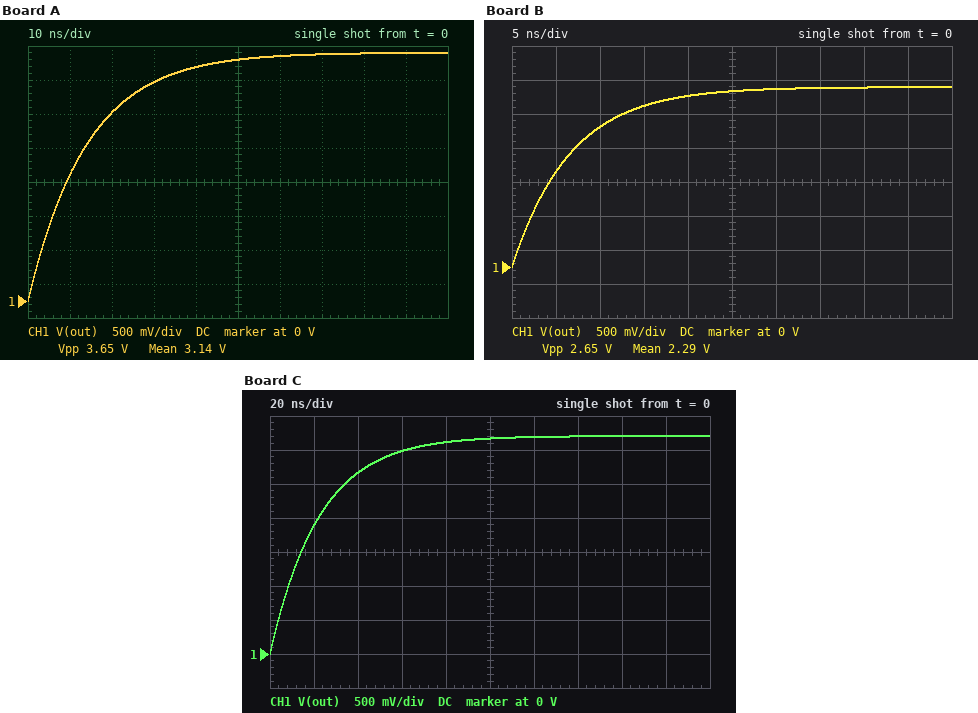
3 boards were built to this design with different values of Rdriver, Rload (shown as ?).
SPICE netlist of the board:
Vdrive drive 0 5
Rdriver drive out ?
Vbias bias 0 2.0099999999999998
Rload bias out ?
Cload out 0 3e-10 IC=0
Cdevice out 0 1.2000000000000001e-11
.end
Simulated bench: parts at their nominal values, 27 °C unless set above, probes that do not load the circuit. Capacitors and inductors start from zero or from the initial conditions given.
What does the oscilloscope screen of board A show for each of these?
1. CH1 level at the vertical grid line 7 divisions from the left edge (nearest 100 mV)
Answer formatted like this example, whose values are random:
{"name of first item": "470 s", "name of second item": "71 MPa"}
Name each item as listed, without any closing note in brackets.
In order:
{"CH1 level at the vertical grid line 7 divisions from the left edge": "3.6 V"}
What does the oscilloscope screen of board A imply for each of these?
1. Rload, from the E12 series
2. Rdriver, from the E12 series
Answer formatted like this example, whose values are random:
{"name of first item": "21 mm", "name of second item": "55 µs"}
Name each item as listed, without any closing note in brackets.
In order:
{"Rload, from the E12 series": "100 Ω", "Rdriver, from the E12 series": "82 Ω"}
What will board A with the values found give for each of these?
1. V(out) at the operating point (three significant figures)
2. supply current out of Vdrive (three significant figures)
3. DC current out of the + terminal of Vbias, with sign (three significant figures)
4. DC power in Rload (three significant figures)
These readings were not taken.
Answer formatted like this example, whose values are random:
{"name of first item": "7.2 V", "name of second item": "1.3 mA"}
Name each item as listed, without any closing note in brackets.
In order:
{"V(out) at the operating point": "3.65 V", "supply current out of Vdrive": "16.4 mA", "DC current out of the + terminal of Vbias, with sign": "-16.4 mA", "DC power in Rload": "27.0 mW"}
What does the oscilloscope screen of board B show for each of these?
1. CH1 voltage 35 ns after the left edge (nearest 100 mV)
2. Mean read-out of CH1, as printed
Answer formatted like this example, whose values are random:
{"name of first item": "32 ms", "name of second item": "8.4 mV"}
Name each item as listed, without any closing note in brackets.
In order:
{"CH1 voltage 35 ns after the left edge": "2.6 V", "Mean read-out of CH1, as printed": "2.29 V"}
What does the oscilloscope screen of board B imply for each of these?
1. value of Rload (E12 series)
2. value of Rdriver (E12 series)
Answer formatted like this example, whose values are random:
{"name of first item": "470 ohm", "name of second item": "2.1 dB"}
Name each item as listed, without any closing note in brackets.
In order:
{"value of Rload": "27 Ω", "value of Rdriver": "100 Ω"}
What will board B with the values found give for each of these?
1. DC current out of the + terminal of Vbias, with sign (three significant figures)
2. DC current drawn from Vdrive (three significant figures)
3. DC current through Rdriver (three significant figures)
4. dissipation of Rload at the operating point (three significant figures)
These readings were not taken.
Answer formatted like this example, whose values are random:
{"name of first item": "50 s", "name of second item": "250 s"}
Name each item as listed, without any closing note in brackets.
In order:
{"DC current out of the + terminal of Vbias, with sign": "-23.5 mA", "DC current drawn from Vdrive": "23.5 mA", "DC current through Rdriver": "23.5 mA", "dissipation of Rload at the operating point": "15.0 mW"}
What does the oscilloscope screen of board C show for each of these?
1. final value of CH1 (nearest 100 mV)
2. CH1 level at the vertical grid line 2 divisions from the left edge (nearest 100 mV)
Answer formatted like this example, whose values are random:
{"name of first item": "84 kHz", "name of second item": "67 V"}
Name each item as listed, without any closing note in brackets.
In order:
{"final value of CH1": "3.2 V", "CH1 level at the vertical grid line 2 divisions from the left edge": "2.7 V"}
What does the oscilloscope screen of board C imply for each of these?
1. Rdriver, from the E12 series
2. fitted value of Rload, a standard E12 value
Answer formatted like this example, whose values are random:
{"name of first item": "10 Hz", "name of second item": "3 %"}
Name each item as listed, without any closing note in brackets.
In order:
{"Rdriver, from the E12 series": "180 Ω", "fitted value of Rload, a standard E12 value": "120 Ω"}
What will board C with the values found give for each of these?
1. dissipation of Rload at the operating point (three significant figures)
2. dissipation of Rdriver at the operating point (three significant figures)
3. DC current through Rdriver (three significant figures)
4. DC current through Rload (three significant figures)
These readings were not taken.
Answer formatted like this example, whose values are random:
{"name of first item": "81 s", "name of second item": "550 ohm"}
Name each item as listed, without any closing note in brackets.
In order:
{"dissipation of Rload at the operating point": "11.9 mW", "dissipation of Rdriver at the operating point": "17.9 mW", "DC current through Rdriver": "9.97 mA", "DC current through Rload": "9.97 mA"}
